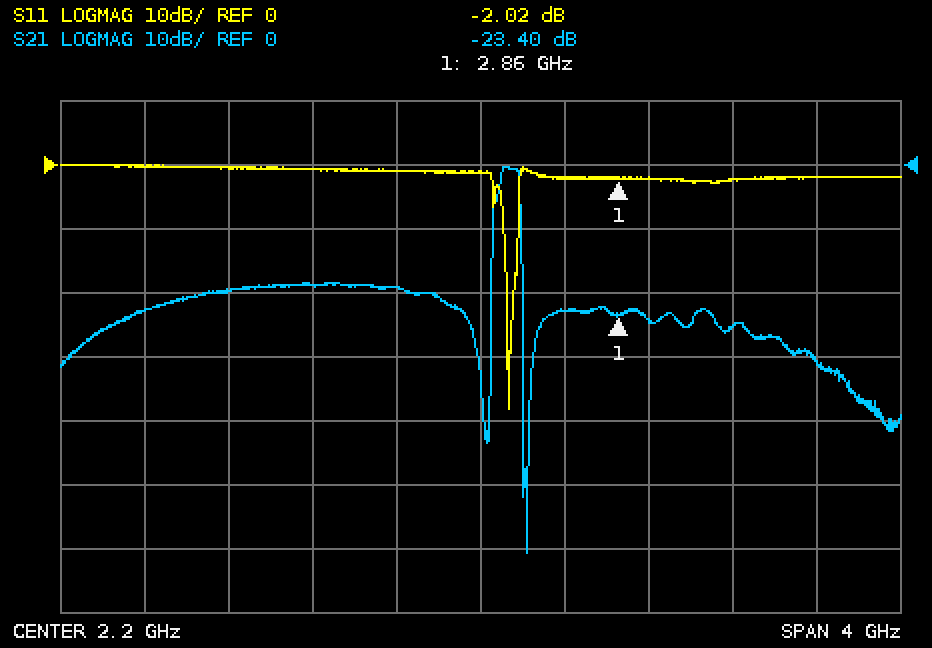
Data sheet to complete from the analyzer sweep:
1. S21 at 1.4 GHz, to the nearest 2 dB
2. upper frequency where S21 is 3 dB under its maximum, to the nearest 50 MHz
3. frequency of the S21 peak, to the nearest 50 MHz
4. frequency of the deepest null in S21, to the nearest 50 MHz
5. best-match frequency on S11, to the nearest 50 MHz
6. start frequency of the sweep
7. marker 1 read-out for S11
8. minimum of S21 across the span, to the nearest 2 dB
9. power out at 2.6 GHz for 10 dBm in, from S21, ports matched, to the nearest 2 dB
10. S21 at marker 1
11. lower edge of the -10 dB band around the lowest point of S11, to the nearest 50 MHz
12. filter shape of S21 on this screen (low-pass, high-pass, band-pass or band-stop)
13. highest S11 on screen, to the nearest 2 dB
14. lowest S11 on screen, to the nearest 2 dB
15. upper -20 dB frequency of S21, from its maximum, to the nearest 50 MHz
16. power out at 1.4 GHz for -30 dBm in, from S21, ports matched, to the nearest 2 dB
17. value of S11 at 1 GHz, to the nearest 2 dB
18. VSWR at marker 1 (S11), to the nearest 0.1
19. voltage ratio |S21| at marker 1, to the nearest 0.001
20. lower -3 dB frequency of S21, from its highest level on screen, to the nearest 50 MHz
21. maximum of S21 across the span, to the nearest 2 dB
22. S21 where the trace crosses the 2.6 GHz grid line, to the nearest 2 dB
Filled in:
-18 dB
2.40 GHz
2.30 GHz
2.40 GHz
2.35 GHz
200 MHz
-2.02 dB
-60 dB
-12 dBm
-23.40 dB
2.30 GHz
band-pass
0 dB
-38 dB
2.40 GHz
-48 dBm
0 dB
8.6
0.068
2.30 GHz
0 dB
-22 dB
